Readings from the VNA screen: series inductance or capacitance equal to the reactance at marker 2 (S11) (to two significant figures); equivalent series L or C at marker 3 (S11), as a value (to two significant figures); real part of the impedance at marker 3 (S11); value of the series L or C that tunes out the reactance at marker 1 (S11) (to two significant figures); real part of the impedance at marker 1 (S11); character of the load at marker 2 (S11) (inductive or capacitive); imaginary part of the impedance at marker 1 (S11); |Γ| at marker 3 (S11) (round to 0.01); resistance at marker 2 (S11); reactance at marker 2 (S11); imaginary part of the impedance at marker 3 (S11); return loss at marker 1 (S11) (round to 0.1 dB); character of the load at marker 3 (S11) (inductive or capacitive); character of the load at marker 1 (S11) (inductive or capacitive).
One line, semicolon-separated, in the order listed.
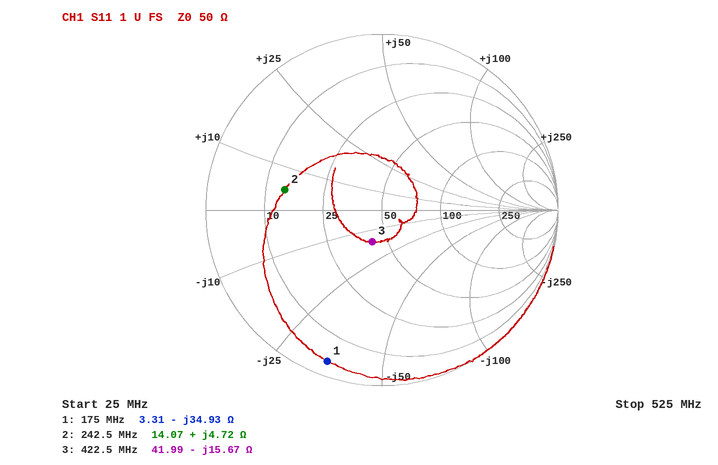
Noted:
3.1 nH; 24 pF; 41.99 Ω; 32 nH; 3.31 Ω; inductive; -34.93 Ω; 0.19; 14.07 Ω; +4.72 Ω; -15.67 Ω; 0.8 dB; capacitive; capacitive
